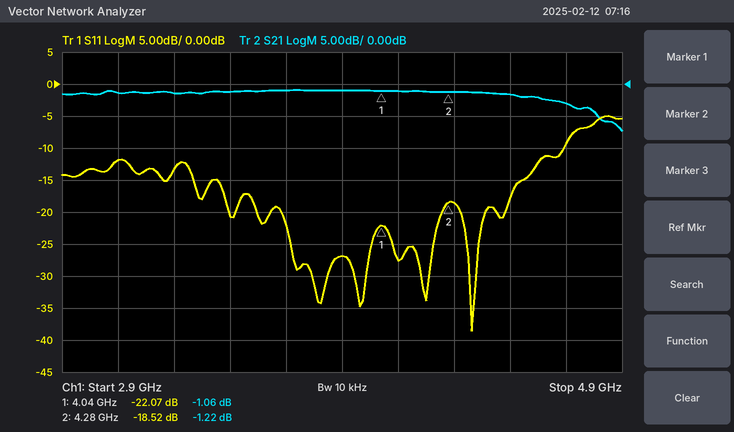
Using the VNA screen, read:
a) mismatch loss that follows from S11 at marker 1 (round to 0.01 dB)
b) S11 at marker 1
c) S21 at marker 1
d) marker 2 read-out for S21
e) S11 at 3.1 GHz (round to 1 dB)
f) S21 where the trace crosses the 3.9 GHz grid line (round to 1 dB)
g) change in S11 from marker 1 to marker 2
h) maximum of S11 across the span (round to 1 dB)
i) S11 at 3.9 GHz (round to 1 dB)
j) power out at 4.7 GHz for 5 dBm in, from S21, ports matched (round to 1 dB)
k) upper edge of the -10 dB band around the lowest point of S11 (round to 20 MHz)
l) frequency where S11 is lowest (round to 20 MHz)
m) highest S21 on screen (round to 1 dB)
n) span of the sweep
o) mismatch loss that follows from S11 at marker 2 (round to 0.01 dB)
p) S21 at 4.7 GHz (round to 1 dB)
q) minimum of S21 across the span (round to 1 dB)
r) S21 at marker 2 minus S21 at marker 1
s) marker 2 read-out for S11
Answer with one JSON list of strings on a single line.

["0.03 dB", "-22.07 dB", "-1.06 dB", "-1.22 dB", "-12 dB", "-1 dB", "3.55 dB", "-5 dB", "-27 dB", "2 dBm", "4.70 GHz", "4.36 GHz", "-1 dB", "2 GHz", "0.06 dB", "-3 dB", "-7 dB", "-0.16 dB", "-18.52 dB"]
